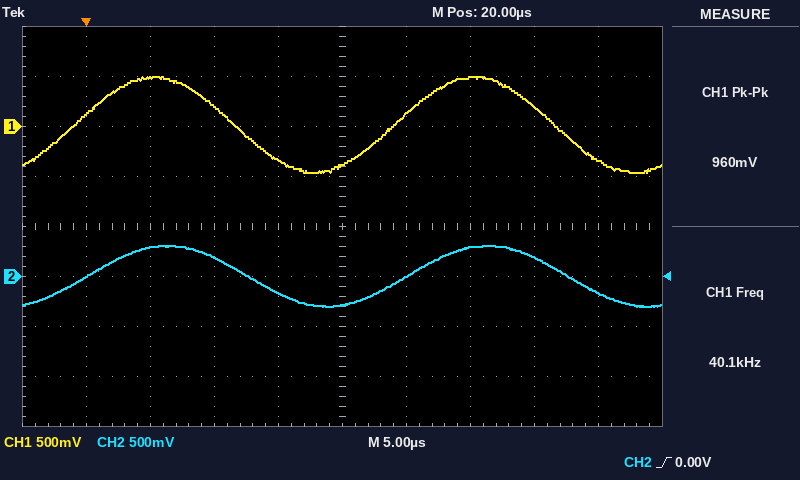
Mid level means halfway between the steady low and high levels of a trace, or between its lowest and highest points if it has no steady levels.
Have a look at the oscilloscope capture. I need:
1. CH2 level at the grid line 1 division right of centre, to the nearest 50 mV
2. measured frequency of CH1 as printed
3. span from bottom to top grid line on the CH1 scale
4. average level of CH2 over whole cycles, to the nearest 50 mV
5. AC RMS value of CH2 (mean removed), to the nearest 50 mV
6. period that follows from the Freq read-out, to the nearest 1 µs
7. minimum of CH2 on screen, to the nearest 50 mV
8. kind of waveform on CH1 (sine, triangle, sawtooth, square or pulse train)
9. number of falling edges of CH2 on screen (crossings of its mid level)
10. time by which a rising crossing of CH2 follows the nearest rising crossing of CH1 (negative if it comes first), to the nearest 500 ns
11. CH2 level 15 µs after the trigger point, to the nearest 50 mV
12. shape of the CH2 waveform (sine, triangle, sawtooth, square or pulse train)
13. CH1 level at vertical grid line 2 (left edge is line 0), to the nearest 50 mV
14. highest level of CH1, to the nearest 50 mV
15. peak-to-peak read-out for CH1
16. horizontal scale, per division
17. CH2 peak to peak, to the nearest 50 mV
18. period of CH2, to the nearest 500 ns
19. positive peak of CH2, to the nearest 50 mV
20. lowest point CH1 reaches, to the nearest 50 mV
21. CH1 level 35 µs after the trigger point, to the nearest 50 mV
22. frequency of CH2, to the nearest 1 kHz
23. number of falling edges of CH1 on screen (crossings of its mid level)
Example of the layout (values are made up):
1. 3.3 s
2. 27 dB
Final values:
1. 0 mV
2. 40.1 kHz
3. 4 V
4. 0 mV
5. 200 mV
6. 25 µs
7. -300 mV
8. sine
9. 2
10. +1.0 µs
11. -150 mV
12. sine
13. 500 mV
14. 500 mV
15. 960 mV
16. 5 µs
17. 600 mV
18. 25.0 µs
19. 300 mV
20. -450 mV
21. 200 mV
22. 40 kHz
23. 2
